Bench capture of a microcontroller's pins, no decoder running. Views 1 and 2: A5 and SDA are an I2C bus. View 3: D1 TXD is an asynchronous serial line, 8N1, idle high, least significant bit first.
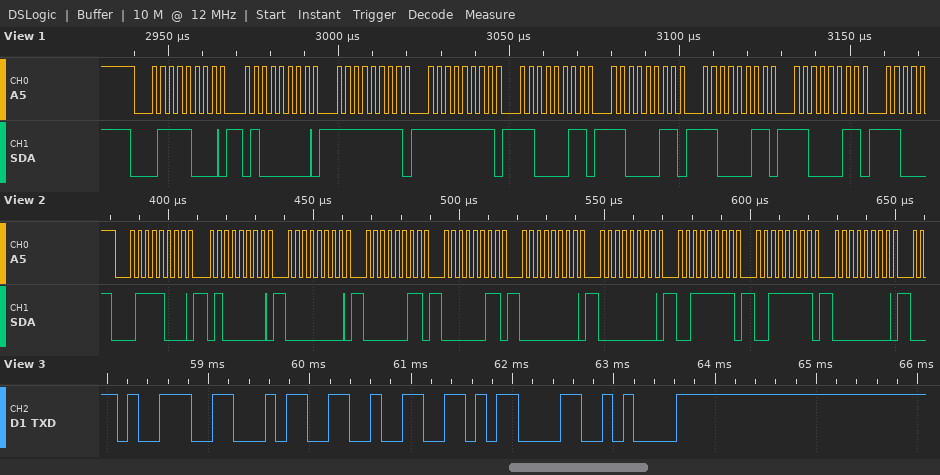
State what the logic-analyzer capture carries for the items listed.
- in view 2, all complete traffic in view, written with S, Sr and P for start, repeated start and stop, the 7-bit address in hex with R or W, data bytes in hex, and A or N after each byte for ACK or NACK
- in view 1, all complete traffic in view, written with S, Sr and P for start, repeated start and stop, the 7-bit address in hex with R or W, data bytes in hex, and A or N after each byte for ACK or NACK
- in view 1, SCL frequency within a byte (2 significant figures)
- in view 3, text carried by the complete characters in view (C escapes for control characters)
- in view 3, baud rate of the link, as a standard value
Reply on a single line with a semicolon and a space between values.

S 3CW A 40 A 00 A 03 A 03 A 00 A 00 A 3F A 3F A 00 A; S 3CW A 40 A FF A FF A C3 A C3 A C3 A C3 A; 400 kHz; "942\r\n"; 9600 baud
